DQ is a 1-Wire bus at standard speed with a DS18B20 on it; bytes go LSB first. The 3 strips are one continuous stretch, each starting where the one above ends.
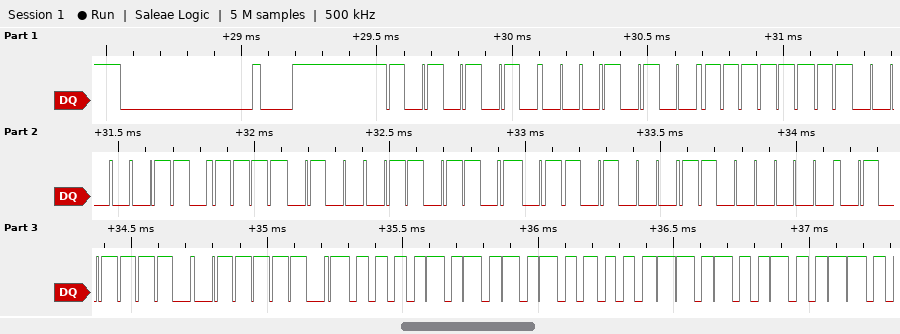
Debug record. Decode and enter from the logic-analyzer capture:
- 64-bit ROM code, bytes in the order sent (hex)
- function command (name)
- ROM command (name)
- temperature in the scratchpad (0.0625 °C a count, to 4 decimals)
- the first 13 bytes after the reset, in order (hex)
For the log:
28 FF 60 2F B6 16 03 7A
Read Scratchpad
Match ROM
85.0000 °C
55 28 FF 60 2F B6 16 03 7A BE 50 05 4B
